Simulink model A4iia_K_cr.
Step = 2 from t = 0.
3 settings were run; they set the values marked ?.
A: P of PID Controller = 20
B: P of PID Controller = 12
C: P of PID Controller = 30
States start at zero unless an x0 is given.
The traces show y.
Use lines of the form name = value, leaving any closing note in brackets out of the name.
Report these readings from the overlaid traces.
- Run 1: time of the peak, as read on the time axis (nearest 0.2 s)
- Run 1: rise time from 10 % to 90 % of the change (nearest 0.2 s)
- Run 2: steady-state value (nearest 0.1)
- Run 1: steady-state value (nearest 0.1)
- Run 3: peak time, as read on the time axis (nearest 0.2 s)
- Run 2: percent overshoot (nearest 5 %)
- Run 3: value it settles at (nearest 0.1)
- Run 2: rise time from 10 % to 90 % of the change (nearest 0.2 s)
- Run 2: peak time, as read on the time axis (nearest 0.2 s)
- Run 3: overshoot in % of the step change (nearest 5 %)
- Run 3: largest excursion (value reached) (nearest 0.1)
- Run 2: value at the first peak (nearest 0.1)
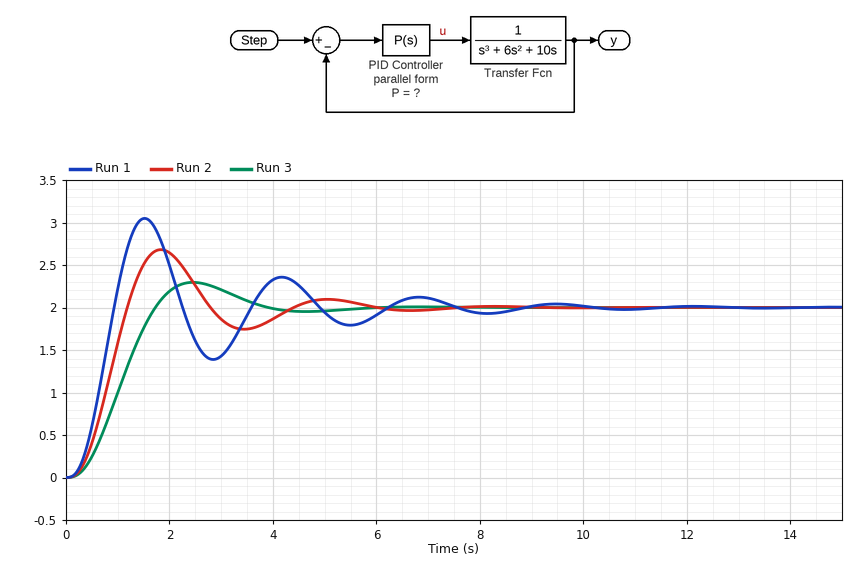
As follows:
Run 1: time of the peak, as read on the time axis = 1.6 s
Run 1: rise time from 10 % to 90 % of the change = 0.6 s
Run 2: steady-state value = 2.0
Run 1: steady-state value = 2.0
Run 3: peak time, as read on the time axis = 2.4 s
Run 2: percent overshoot = 35 %
Run 3: value it settles at = 2.0
Run 2: rise time from 10 % to 90 % of the change = 0.8 s
Run 2: peak time, as read on the time axis = 1.8 s
Run 3: overshoot in % of the step change = 15 %
Run 3: largest excursion (value reached) = 2.3
Run 2: value at the first peak = 2.7
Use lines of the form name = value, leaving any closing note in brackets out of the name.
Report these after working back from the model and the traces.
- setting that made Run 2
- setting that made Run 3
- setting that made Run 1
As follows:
setting that made Run 2 = A
setting that made Run 3 = B
setting that made Run 1 = C
